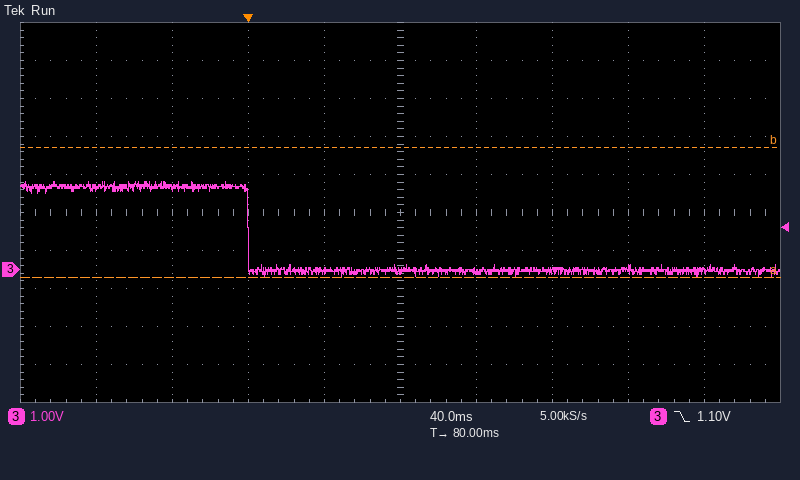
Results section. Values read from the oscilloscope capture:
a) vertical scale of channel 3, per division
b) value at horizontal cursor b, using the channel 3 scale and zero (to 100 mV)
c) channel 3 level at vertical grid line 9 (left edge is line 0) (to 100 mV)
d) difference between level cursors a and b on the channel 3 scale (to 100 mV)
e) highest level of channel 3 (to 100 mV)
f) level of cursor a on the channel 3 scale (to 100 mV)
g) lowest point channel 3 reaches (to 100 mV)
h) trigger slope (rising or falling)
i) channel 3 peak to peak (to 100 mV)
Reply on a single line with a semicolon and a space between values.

1 V; 3.2 V; 0.0 V; 3.4 V; 2.3 V; -200 mV; -200 mV; falling; 2.5 V
